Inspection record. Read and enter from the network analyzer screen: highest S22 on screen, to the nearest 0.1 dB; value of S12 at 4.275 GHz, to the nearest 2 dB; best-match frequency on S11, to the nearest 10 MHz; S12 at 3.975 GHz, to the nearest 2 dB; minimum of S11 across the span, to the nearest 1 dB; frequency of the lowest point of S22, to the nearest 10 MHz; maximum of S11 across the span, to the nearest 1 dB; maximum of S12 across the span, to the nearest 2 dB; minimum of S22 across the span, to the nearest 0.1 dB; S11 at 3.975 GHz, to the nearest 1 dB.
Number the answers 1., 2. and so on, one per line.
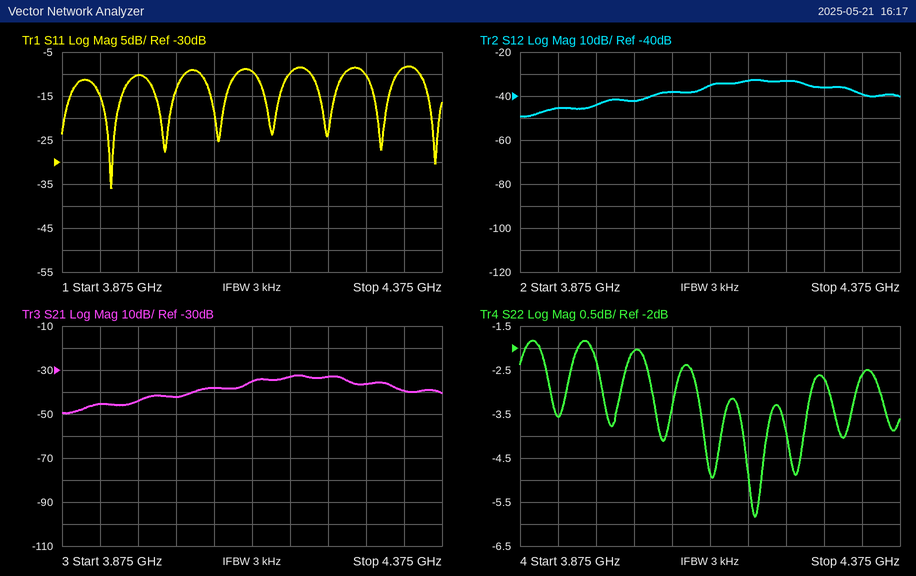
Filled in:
1. -1.8 dB
2. -36 dB
3. 3.94 GHz
4. -44 dB
5. -36 dB
6. 4.18 GHz
7. -8 dB
8. -32 dB
9. -5.8 dB
10. -10 dB
